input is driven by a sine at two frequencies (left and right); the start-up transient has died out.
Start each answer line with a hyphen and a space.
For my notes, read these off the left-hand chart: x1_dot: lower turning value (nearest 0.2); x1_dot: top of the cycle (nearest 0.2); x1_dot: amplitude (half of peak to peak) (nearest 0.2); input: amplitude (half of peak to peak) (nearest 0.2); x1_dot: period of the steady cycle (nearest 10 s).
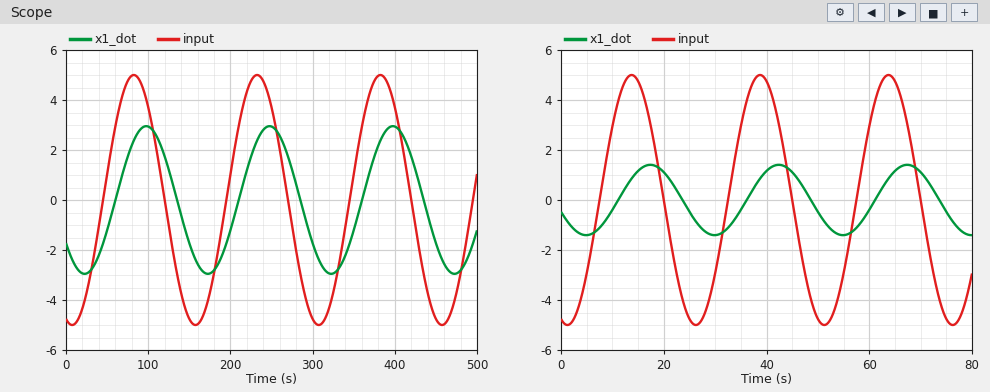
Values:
- -3.0
- 3.0
- 3.0
- 5.0
- 150 s
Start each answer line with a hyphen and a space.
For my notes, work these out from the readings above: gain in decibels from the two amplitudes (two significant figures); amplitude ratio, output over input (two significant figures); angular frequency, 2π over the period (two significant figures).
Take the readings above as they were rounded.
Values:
- -4.4 dB
- 0.60
- 0.042 rad/s
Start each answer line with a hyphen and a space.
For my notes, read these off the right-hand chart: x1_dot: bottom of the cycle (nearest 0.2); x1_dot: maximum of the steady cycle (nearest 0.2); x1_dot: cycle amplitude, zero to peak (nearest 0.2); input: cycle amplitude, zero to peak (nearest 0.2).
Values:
- -1.4
- 1.4
- 1.4
- 5.0
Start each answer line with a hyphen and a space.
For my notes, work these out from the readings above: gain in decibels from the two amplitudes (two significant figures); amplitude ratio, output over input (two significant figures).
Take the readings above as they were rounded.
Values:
- -11 dB
- 0.28
